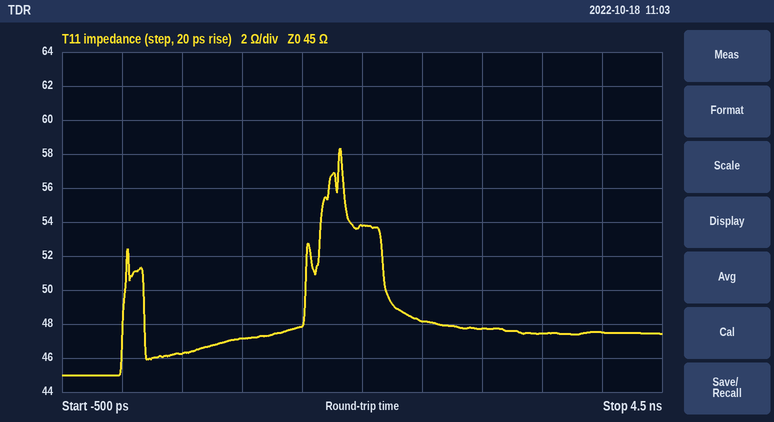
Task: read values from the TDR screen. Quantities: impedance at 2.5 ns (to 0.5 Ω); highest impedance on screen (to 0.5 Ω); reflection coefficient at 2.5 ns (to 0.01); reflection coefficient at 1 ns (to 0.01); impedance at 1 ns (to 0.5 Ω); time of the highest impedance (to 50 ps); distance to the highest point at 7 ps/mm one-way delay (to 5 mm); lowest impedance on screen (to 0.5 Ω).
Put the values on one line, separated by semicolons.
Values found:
48.0 Ω; 58.5 Ω; +0.03; +0.02; 47.0 Ω; 1.80 ns; 130 mm; 45.0 Ω
